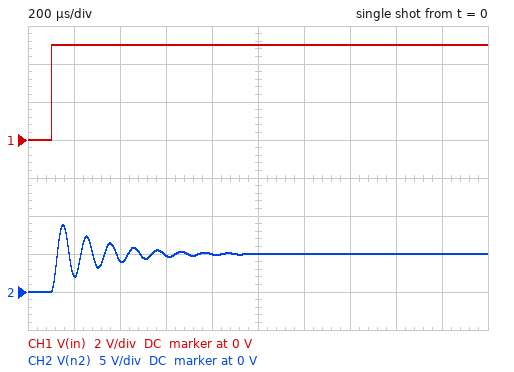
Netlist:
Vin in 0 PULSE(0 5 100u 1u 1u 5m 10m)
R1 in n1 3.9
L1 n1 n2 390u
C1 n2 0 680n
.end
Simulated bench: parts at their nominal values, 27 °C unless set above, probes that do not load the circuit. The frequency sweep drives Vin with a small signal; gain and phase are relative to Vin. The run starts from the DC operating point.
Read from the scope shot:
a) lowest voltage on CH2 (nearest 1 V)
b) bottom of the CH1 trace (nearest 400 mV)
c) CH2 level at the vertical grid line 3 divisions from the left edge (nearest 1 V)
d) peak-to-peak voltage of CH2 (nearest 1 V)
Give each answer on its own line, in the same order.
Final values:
0 V
0 V
5 V
9 V
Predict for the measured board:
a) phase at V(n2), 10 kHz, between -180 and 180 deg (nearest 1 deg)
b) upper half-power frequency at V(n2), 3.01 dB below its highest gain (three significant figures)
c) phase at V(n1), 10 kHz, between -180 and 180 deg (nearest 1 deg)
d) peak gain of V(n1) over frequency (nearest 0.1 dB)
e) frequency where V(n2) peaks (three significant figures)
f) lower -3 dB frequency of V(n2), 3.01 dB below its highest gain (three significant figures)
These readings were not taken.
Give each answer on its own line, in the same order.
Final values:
-106 deg
10.5 kHz
74 deg
0 dB
9.71 kHz
8.87 kHz
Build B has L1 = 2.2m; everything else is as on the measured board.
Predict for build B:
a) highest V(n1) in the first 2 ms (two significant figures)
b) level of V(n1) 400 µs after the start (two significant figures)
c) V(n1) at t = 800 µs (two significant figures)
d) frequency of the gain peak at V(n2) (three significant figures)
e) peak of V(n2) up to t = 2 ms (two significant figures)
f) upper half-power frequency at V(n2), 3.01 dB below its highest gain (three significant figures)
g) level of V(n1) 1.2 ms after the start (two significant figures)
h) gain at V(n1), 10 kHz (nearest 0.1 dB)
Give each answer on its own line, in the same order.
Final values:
5.3 V
4.7 V
5.1 V
4.11 kHz
9.5 V
4.25 kHz
5.0 V
0 dB
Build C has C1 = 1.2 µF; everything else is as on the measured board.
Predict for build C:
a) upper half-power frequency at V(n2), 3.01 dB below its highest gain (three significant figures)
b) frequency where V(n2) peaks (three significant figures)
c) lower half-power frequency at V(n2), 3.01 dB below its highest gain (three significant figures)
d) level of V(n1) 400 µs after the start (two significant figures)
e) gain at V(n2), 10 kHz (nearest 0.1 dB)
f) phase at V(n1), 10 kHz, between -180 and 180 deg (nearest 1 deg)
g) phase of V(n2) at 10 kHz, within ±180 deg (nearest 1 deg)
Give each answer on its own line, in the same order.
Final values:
8.03 kHz
7.27 kHz
6.42 kHz
4.8 V
0.9 dB
19 deg
-161 deg
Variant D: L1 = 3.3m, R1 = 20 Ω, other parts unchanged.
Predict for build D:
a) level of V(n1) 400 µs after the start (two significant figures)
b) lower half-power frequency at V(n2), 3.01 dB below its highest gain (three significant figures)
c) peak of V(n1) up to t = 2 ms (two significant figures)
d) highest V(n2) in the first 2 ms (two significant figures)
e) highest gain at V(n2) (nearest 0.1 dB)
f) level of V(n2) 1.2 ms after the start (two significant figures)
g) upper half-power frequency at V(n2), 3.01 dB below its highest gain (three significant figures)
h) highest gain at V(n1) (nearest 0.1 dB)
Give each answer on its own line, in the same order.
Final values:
5.0 V
2.76 kHz
5.7 V
8.2 V
10.9 dB
5.1 V
3.75 kHz
0 dB
